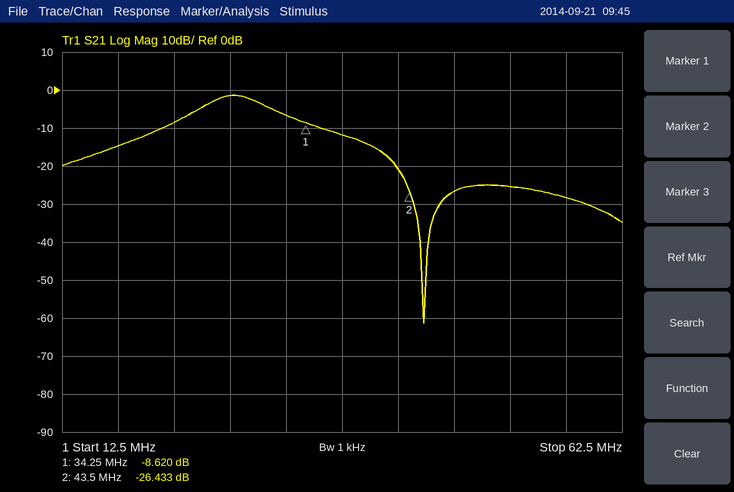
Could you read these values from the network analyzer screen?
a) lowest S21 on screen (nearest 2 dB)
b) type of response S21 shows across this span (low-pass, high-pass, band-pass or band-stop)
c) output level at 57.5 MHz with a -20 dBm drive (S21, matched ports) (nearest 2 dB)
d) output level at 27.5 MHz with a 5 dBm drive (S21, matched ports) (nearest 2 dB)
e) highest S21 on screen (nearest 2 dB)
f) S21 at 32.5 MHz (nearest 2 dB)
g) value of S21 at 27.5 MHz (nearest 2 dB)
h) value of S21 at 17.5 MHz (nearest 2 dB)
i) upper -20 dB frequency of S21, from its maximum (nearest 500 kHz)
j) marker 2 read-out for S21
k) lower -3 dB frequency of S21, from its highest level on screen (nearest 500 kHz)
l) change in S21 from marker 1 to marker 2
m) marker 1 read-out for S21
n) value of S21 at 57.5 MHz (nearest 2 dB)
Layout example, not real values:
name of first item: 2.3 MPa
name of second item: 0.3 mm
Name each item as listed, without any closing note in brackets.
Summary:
lowest S21 on screen: -62 dB
type of response S21 shows across this span: band-pass
output level at 57.5 MHz with a -20 dBm drive (S21, matched ports): -48 dBm
output level at 27.5 MHz with a 5 dBm drive (S21, matched ports): 4 dBm
highest S21 on screen: -2 dB
S21 at 32.5 MHz: -6 dB
value of S21 at 27.5 MHz: -2 dB
value of S21 at 17.5 MHz: -14 dB
upper -20 dB frequency of S21, from its maximum: 42.5 MHz
marker 2 read-out for S21: -26.433 dB
lower -3 dB frequency of S21, from its highest level on screen: 25.0 MHz
change in S21 from marker 1 to marker 2: -17.813 dB
marker 1 read-out for S21: -8.620 dB
value of S21 at 57.5 MHz: -28 dB
